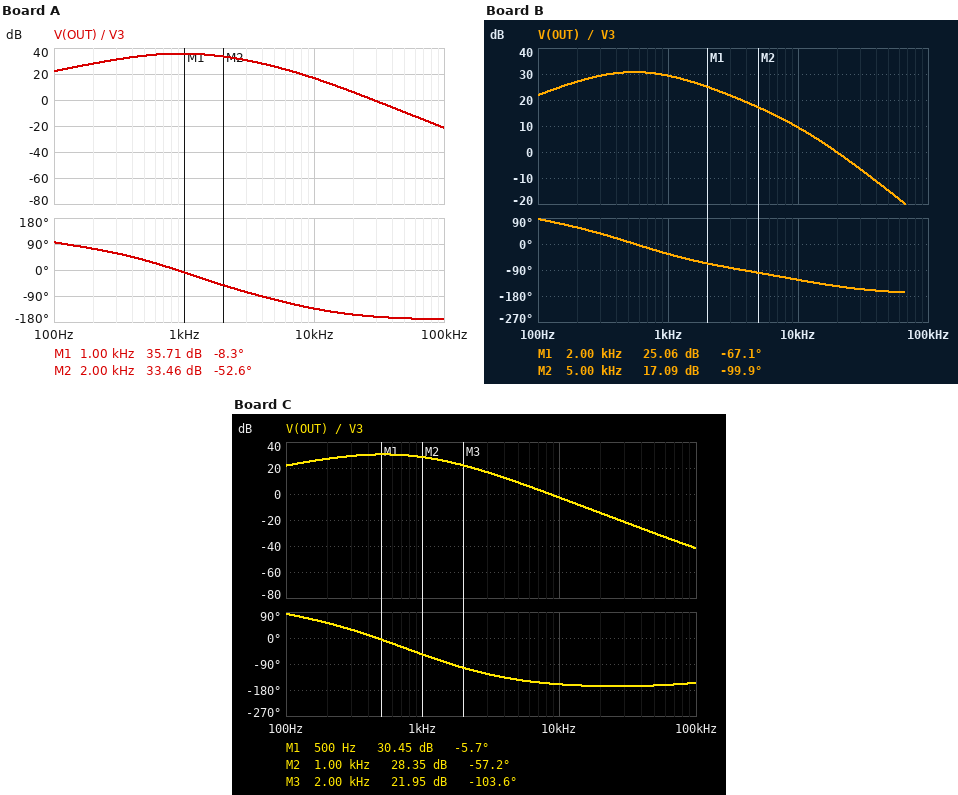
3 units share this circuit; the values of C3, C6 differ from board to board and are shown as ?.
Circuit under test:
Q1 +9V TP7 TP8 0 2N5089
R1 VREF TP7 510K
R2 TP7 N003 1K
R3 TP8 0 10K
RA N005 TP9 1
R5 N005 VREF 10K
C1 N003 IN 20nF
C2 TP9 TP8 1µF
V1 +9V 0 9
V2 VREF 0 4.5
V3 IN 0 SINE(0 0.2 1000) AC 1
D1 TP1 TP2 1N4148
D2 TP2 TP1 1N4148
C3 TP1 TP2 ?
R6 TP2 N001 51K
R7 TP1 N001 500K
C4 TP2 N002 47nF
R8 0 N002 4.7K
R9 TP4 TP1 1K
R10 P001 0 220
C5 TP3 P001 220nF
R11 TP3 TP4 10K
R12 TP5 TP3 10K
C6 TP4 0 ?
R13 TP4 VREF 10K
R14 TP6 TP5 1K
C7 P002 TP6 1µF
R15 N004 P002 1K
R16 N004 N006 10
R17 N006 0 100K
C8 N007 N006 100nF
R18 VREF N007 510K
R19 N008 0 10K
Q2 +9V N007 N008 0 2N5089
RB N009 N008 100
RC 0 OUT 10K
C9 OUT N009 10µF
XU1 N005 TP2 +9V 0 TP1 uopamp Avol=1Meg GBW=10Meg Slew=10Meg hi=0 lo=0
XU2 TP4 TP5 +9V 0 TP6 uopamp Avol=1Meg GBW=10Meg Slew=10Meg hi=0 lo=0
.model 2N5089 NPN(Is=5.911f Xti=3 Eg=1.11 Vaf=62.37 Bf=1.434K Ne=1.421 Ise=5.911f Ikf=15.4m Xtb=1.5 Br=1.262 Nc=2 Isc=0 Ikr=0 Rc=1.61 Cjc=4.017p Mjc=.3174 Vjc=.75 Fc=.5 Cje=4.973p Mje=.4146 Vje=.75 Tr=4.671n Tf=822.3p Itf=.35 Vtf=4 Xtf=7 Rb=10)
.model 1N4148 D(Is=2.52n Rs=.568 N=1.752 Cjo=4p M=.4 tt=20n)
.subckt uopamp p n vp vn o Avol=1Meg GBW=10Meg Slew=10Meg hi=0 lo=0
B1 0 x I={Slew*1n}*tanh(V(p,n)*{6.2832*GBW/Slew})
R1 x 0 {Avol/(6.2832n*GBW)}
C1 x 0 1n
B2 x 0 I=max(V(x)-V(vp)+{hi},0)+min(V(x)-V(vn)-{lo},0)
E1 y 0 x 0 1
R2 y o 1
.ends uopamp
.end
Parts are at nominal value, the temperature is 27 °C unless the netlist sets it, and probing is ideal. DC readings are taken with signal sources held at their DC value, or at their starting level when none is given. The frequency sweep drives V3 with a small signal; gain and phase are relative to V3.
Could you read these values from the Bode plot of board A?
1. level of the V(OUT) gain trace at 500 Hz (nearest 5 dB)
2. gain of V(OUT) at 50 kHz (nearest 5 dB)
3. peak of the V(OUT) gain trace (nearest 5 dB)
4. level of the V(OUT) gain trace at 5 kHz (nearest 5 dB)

35 dB
-10 dB
35 dB
25 dB
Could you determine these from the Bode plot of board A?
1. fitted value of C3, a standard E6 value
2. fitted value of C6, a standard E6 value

33 pF
150 nF
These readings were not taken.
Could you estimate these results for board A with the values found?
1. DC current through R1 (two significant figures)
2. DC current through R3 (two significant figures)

460 nA
360 µA
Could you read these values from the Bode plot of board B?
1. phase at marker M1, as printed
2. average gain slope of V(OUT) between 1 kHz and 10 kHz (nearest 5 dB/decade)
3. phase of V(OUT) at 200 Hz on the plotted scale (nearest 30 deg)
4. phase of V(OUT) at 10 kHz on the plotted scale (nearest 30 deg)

-67.1 deg
-20 dB/decade
60 deg
-120 deg
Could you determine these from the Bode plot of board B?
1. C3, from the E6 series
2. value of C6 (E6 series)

15 pF
470 nF
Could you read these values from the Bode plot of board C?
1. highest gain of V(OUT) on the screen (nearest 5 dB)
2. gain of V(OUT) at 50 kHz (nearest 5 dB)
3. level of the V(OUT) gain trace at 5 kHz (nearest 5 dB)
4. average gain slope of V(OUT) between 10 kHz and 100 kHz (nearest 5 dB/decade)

30 dB
-30 dB
10 dB
-40 dB/decade
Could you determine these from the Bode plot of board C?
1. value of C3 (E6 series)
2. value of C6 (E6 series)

150 pF
470 nF
